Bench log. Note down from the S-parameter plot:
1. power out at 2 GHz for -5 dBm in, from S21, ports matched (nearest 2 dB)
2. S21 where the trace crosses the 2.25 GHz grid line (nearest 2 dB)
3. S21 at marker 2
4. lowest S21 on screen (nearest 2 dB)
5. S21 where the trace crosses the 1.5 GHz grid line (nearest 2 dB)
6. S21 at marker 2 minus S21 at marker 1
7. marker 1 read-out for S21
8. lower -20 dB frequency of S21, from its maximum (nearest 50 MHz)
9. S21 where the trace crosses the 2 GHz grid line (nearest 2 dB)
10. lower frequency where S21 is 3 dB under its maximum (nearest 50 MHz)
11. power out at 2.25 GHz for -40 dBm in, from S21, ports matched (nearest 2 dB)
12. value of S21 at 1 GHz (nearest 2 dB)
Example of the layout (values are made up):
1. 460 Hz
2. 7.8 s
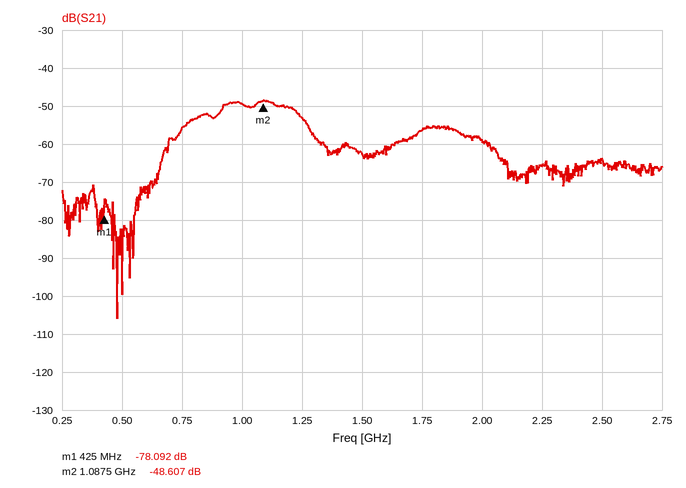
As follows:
1. -64 dBm
2. -66 dB
3. -48.607 dB
4. -106 dB
5. -62 dB
6. 29.485 dB
7. -78.092 dB
8. 650 MHz
9. -60 dB
10. 900 MHz
11. -106 dBm
12. -50 dB
